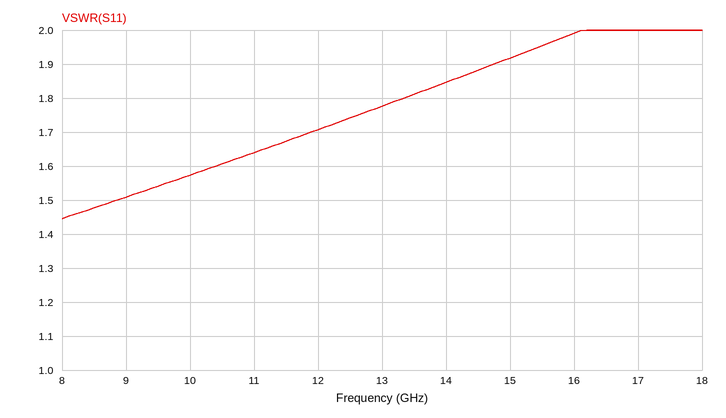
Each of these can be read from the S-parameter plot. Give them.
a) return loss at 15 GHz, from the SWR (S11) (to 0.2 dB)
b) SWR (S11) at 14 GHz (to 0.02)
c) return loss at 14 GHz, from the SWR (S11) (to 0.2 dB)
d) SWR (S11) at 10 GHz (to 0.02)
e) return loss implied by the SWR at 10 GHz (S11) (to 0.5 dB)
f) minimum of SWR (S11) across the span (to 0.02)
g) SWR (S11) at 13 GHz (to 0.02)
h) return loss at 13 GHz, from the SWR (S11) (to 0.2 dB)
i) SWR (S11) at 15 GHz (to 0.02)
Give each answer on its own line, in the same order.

10.0 dB
1.84
10.6 dB
1.58
13.0 dB
1.44
1.78
11.0 dB
1.92
